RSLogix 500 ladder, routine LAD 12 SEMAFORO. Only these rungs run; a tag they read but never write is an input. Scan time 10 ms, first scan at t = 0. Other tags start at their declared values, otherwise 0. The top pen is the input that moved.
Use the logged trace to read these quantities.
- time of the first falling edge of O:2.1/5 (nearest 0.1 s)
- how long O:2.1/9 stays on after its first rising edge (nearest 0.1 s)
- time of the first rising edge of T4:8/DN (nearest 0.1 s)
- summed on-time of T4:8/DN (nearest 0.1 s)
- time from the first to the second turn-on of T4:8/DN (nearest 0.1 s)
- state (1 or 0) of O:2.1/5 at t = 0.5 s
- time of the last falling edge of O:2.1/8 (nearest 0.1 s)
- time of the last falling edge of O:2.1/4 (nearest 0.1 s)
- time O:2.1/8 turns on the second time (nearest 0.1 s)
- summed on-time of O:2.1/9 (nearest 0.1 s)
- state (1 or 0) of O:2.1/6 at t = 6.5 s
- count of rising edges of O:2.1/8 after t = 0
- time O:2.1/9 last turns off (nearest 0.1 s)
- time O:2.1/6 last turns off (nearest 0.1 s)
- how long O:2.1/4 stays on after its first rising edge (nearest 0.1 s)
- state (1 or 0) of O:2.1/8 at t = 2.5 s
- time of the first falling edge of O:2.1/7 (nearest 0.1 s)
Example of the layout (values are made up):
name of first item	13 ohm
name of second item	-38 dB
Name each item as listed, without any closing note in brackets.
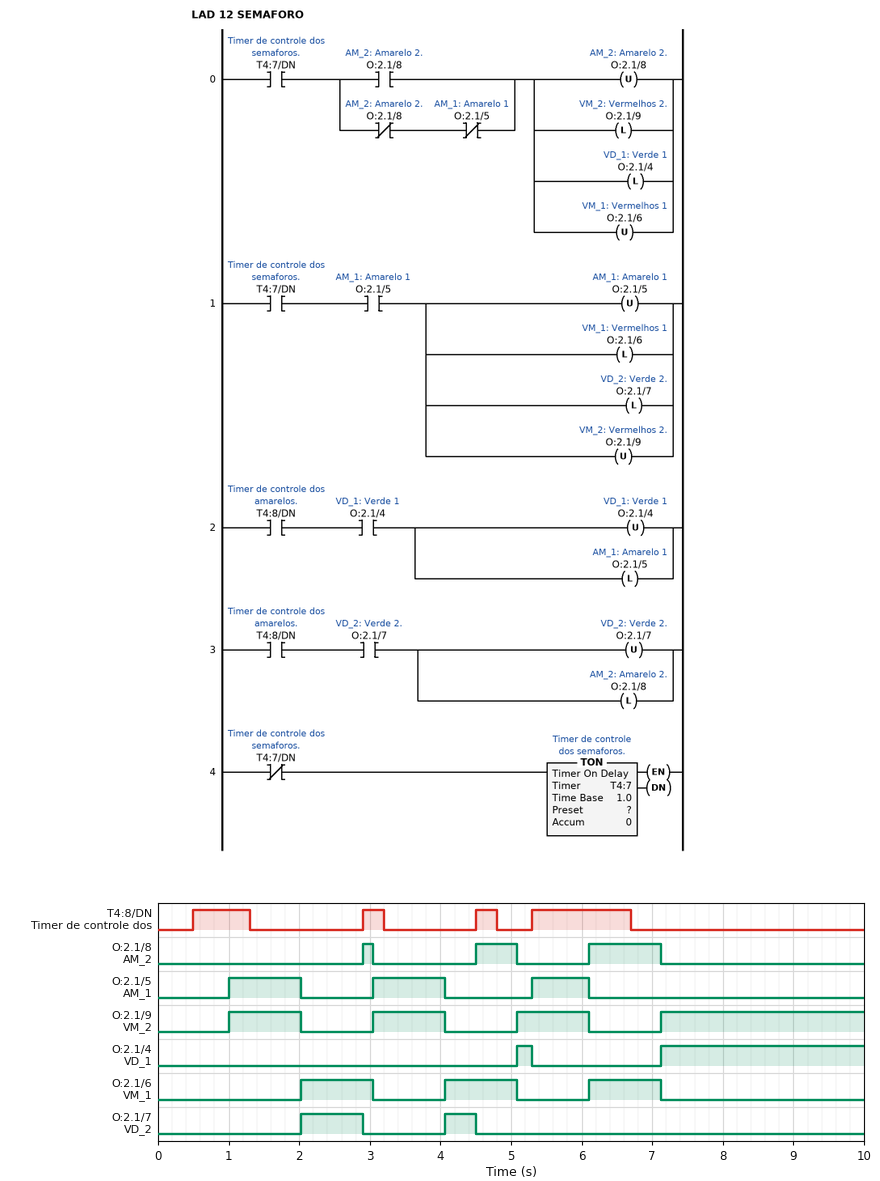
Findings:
time of the first falling edge of O:2.1/5	2.0 s
how long O:2.1/9 stays on after its first rising edge	1.0 s
time of the first rising edge of T4:8/DN	0.5 s
summed on-time of T4:8/DN	2.8 s
time from the first to the second turn-on of T4:8/DN	2.4 s
state (1 or 0) of O:2.1/5 at t = 0.5 s	0
time of the last falling edge of O:2.1/8	7.1 s
time of the last falling edge of O:2.1/4	5.3 s
time O:2.1/8 turns on the second time	4.5 s
summed on-time of O:2.1/9	5.9 s
state (1 or 0) of O:2.1/6 at t = 6.5 s	1
count of rising edges of O:2.1/8 after t = 0	3
time O:2.1/9 last turns off	6.1 s
time O:2.1/6 last turns off	7.1 s
how long O:2.1/4 stays on after its first rising edge	0.2 s
state (1 or 0) of O:2.1/8 at t = 2.5 s	0
time of the first falling edge of O:2.1/7	2.9 s
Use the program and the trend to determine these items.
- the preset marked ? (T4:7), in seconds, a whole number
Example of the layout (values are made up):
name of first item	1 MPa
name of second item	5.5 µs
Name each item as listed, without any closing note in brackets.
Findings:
the preset marked ? (T4:7), in seconds, a whole number	1 s
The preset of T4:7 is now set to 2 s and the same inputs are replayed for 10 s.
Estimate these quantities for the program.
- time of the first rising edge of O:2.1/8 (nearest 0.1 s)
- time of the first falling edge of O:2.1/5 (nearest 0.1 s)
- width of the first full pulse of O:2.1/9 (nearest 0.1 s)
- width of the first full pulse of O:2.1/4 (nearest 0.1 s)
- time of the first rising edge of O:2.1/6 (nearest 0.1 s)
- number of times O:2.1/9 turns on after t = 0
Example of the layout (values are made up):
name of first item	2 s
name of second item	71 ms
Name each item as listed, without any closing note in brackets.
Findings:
time of the first rising edge of O:2.1/8	4.5 s
time of the first falling edge of O:2.1/5	4.0 s
width of the first full pulse of O:2.1/9	2.0 s
width of the first full pulse of O:2.1/4	0.9 s
time of the first rising edge of O:2.1/6	4.0 s
number of times O:2.1/9 turns on after t = 0	2
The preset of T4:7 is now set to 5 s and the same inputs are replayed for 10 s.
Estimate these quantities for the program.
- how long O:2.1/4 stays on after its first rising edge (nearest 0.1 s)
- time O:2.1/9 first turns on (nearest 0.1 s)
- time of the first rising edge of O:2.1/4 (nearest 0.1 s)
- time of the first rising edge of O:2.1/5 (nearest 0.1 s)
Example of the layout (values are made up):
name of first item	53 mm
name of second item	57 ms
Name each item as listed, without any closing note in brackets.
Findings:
how long O:2.1/4 stays on after its first rising edge	0.3 s
time O:2.1/9 first turns on	5.0 s
time of the first rising edge of O:2.1/4	5.0 s
time of the first rising edge of O:2.1/5	5.3 s
